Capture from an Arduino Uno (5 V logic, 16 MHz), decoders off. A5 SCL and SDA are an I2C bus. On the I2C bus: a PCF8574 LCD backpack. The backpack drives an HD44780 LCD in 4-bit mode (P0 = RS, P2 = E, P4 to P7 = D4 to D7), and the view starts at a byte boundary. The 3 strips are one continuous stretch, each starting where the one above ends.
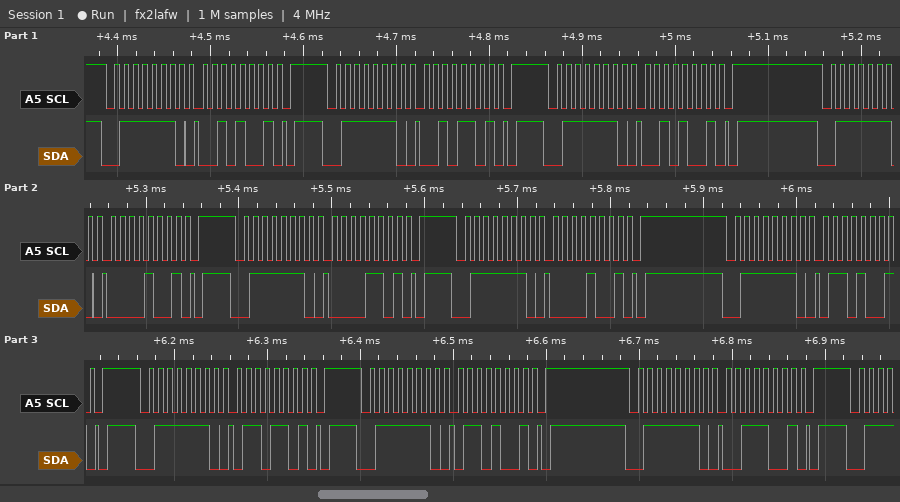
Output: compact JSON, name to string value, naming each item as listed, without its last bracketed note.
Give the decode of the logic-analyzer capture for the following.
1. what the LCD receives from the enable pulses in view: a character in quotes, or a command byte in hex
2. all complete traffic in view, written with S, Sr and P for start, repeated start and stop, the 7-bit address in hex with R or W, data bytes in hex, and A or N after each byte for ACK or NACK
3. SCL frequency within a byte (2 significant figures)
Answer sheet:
{"what the LCD receives from the enable pulses in view: a character in quotes, or a command byte in hex": "' '", "all complete traffic in view, written with S, Sr and P for start, repeated start and stop, the 7-bit address in hex with R or W, data bytes in hex, and A or N after each byte for ACK or NACK": "S 3FW A 29 A P S 3FW A 2D A P S 3FW A 29 A P S 3FW A 09 A P S 3FW A 0D A P S 3FW A 09 A P S 3FW A 69 A P S 3FW A 6D A P S 3FW A 69 A P S 3FW A 39 A P", "SCL frequency within a byte": "100 kHz"}
